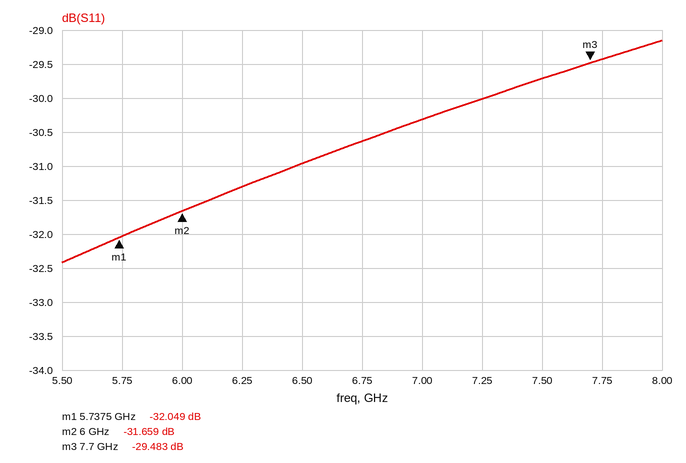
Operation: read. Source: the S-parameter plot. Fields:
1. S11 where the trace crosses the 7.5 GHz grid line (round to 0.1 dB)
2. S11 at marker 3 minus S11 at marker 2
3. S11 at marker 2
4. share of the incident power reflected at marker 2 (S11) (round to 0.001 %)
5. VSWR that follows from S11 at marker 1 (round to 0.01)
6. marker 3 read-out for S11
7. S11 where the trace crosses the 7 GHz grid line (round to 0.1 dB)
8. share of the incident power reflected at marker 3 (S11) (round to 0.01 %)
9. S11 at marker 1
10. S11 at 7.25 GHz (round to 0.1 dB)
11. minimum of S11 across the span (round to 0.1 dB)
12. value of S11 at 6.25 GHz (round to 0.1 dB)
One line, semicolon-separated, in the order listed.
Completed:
-29.7 dB; 2.176 dB; -31.659 dB; 0.068 %; 1.05; -29.483 dB; -30.3 dB; 0.11 %; -32.049 dB; -30.0 dB; -32.4 dB; -31.3 dB
